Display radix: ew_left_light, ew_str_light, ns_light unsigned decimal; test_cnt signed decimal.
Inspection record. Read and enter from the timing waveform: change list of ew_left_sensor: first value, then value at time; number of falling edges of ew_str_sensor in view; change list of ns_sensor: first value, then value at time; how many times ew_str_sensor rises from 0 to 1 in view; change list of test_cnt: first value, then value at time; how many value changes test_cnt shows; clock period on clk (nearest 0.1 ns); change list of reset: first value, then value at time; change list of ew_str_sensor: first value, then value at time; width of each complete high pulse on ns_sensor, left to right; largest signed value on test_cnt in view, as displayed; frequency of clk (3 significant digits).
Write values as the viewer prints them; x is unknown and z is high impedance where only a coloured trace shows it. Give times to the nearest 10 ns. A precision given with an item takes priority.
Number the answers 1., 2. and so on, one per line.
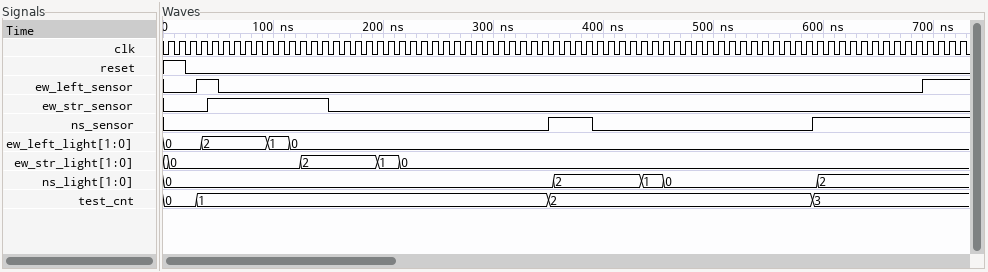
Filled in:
1. 0, 1 at 30 ns, 0 at 50 ns, 1 at 690 ns
2. 1
3. 0, 1 at 350 ns, 0 at 390 ns, 1 at 590 ns
4. 1
5. 0, 1 at 30 ns, 2 at 350 ns, 3 at 590 ns
6. 3
7. 10 ns
8. 1, 0 at 20 ns
9. 0, 1 at 40 ns, 0 at 150 ns
10. 40 ns
11. 3
12. 100 MHz
